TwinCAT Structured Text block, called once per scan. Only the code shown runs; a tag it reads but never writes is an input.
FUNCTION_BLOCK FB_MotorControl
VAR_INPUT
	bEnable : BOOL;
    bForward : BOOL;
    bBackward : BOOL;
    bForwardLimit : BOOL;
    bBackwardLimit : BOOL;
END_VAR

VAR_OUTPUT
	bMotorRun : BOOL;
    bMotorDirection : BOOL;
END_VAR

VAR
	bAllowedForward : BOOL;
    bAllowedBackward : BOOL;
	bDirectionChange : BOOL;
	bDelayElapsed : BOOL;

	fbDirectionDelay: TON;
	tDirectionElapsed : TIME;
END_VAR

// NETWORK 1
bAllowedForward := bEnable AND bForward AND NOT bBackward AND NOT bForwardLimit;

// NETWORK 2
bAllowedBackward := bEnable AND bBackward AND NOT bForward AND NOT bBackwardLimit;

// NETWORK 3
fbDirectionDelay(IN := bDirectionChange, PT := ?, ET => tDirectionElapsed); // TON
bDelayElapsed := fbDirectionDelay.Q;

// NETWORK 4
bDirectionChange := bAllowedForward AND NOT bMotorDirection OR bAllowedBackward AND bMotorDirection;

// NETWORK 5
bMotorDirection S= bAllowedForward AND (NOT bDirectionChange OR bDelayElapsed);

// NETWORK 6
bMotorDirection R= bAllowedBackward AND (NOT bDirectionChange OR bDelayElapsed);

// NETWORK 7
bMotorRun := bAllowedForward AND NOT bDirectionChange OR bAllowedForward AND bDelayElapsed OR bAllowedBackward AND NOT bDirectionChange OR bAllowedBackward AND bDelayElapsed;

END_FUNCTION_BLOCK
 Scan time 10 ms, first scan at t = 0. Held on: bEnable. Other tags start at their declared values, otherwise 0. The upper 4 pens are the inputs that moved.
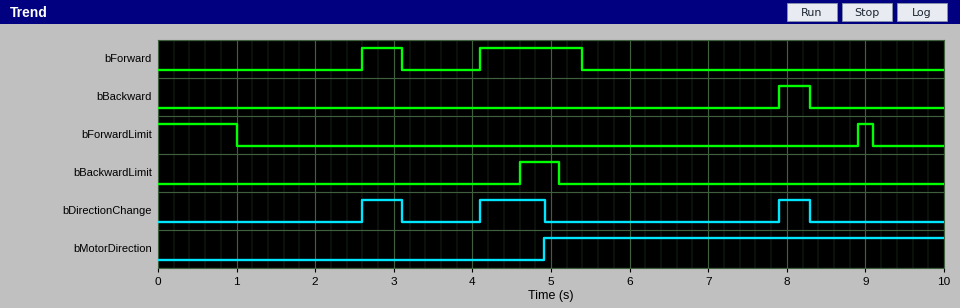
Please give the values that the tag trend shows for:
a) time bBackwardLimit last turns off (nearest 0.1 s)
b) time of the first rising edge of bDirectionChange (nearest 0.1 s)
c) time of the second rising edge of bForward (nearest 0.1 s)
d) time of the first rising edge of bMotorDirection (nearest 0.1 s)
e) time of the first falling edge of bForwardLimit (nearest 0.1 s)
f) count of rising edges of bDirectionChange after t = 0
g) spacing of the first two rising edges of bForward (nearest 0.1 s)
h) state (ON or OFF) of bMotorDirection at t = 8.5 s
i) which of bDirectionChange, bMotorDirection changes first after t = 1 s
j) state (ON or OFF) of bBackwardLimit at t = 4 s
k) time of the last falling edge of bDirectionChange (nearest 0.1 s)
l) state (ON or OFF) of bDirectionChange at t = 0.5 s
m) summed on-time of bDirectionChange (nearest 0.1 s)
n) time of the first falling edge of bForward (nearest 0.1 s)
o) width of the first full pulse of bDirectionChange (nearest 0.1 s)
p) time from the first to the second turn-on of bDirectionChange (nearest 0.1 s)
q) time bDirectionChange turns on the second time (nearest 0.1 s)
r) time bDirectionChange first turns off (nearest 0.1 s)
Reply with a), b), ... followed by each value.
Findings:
a) 5.1 s
b) 2.6 s
c) 4.1 s
d) 4.9 s
e) 1.0 s
f) 3
g) 1.5 s
h) ON
i) bDirectionChange
j) OFF
k) 8.3 s
l) OFF
m) 1.7 s
n) 3.1 s
o) 0.5 s
p) 1.5 s
q) 4.1 s
r) 3.1 s
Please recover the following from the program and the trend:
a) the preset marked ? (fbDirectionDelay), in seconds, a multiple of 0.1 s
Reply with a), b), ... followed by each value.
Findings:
a) 0.8 s
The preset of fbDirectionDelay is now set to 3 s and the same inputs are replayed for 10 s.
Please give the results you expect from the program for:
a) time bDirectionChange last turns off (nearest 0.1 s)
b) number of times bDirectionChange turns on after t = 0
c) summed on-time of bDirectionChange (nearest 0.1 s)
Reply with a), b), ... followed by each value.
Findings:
a) 5.4 s
b) 2
c) 1.8 s
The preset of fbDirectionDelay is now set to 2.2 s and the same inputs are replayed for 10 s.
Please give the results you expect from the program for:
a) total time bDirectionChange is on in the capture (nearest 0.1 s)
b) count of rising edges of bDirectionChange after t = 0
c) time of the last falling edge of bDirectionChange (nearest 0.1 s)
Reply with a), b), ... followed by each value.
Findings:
a) 1.8 s
b) 2
c) 5.4 s
